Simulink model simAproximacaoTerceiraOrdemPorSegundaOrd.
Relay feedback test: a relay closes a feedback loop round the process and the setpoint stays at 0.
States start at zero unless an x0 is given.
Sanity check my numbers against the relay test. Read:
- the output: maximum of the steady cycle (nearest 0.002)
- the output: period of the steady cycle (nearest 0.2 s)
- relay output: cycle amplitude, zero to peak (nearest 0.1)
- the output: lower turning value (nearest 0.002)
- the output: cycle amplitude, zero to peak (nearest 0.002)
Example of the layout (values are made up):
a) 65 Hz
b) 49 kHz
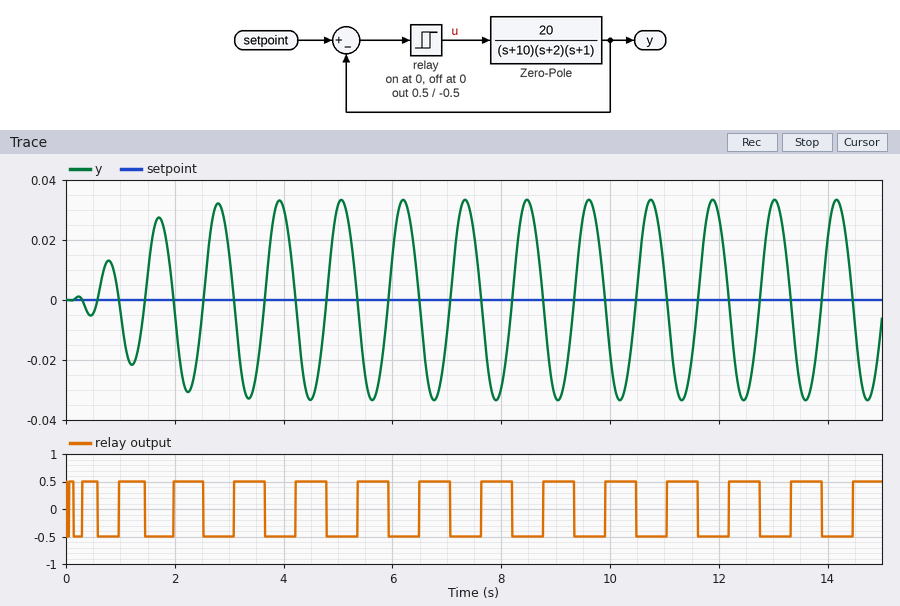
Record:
a) 0.034
b) 1.2 s
c) 0.5
d) -0.034
e) 0.034
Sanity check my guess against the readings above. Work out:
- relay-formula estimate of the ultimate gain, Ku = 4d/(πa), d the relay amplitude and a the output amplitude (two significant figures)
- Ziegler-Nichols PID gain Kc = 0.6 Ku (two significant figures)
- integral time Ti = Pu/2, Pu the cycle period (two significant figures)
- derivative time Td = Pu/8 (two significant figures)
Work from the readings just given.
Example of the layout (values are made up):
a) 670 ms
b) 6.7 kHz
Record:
a) 19
b) 11
c) 0.60 s
d) 0.15 s
